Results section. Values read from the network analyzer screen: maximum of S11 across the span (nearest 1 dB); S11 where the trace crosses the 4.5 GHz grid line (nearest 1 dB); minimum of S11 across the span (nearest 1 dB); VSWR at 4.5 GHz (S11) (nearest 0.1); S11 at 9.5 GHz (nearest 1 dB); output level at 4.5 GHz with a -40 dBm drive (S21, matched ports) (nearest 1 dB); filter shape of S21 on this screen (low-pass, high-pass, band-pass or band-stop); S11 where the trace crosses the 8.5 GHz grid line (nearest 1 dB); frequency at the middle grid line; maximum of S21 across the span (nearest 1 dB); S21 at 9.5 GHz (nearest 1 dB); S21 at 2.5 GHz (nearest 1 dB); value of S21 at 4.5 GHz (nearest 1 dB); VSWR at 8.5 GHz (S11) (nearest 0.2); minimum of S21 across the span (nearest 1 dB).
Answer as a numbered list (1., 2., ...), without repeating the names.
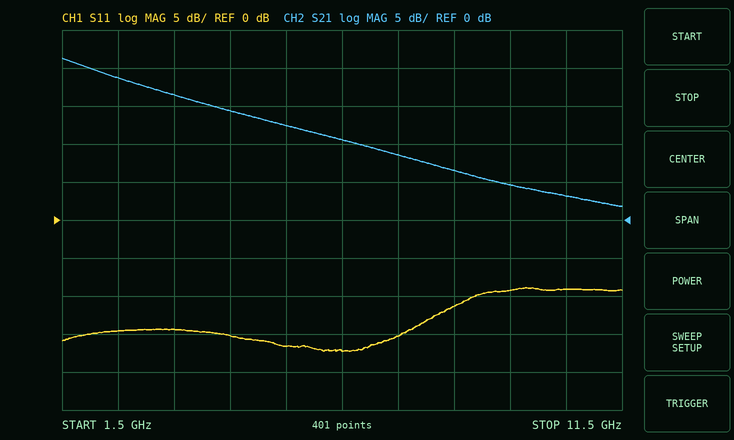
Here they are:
1. -9 dB
2. -15 dB
3. -17 dB
4. 1.4
5. -9 dB
6. -26 dBm
7. low-pass
8. -11 dB
9. 6.5 GHz
10. 21 dB
11. 5 dB
12. 19 dB
13. 14 dB
14. 1.8
15. 2 dB
